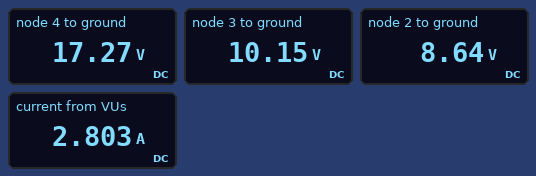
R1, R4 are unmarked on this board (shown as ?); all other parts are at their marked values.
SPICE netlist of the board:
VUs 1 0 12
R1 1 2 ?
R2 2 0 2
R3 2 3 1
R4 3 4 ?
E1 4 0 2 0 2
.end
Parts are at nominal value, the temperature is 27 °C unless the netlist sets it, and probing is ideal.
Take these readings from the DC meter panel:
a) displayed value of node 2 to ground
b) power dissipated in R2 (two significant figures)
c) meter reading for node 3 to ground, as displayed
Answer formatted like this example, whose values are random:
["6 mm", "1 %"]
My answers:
["8.64 V", "37 W", "10.15 V"]
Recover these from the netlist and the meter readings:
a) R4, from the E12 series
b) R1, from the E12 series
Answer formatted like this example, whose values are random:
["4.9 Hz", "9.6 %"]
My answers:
["4.7 Ω", "1.2 Ω"]
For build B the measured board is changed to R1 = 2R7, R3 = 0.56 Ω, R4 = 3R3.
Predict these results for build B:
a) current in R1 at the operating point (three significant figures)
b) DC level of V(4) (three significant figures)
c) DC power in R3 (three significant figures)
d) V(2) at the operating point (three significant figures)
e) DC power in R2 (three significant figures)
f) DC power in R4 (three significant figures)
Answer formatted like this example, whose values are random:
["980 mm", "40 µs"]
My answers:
["1.75 A", "14.5 V", "1.99 W", "7.27 V", "26.4 W", "11.7 W"]
